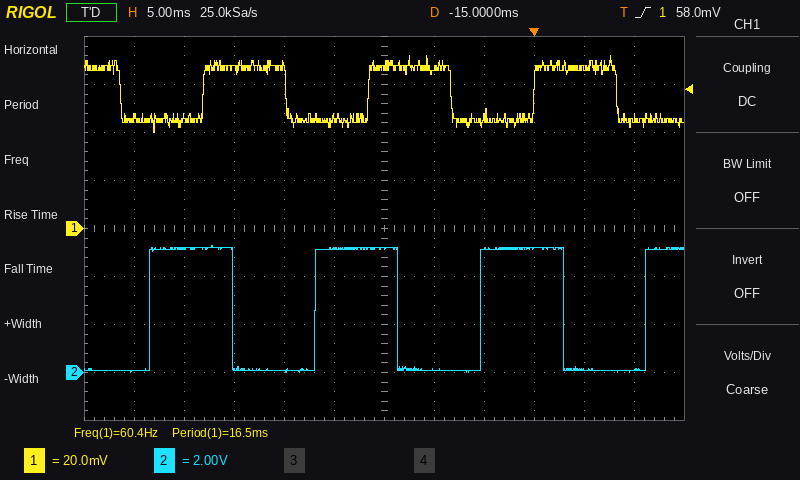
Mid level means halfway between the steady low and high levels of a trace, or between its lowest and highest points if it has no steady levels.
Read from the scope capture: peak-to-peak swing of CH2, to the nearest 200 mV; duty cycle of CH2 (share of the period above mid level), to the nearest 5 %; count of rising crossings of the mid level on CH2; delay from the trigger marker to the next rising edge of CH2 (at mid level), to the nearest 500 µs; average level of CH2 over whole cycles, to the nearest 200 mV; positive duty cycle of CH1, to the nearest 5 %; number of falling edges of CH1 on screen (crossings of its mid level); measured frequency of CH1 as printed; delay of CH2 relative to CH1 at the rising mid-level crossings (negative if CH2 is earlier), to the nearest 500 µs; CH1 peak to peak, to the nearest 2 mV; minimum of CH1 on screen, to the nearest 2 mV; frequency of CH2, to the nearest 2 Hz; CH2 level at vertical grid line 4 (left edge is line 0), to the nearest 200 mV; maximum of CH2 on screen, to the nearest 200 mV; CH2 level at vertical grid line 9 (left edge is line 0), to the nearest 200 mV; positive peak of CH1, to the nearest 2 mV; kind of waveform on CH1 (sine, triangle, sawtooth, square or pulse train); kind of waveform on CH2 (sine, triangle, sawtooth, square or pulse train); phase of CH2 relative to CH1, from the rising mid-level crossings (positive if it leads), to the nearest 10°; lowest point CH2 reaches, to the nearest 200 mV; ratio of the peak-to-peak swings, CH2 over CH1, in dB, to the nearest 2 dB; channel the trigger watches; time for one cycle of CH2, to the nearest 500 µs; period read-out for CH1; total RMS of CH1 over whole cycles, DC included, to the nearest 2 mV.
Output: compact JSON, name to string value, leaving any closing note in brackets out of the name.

{"peak-to-peak swing of CH2, to the nearest 200 mV": "5.2 V", "duty cycle of CH2 (share of the period above mid level), to the nearest 5 %": "50 %", "count of rising crossings of the mid level on CH2": "4", "delay from the trigger marker to the next rising edge of CH2 (at mid level), to the nearest 500 µs": "11.0 ms", "average level of CH2 over whole cycles, to the nearest 200 mV": "2.6 V", "positive duty cycle of CH1, to the nearest 5 %": "50 %", "number of falling edges of CH1 on screen": "4", "measured frequency of CH1 as printed": "60.4 Hz", "delay of CH2 relative to CH1 at the rising mid-level crossings (negative if CH2 is earlier), to the nearest 500 µs": "-5.5 ms", "CH1 peak to peak, to the nearest 2 mV": "32 mV", "minimum of CH1 on screen, to the nearest 2 mV": "40 mV", "frequency of CH2, to the nearest 2 Hz": "60 Hz", "CH2 level at vertical grid line 4 (left edge is line 0), to the nearest 200 mV": "0.0 V", "maximum of CH2 on screen, to the nearest 200 mV": "5.2 V", "CH2 level at vertical grid line 9 (left edge is line 0), to the nearest 200 mV": "5.2 V", "positive peak of CH1, to the nearest 2 mV": "72 mV", "kind of waveform on CH1": "square", "kind of waveform on CH2": "square", "phase of CH2 relative to CH1, from the rising mid-level crossings (positive if it leads), to the nearest 10°": "+120°", "lowest point CH2 reaches, to the nearest 200 mV": "0.0 V", "ratio of the peak-to-peak swings, CH2 over CH1, in dB, to the nearest 2 dB": "44 dB", "channel the trigger watches": "CH1", "time for one cycle of CH2, to the nearest 500 µs": "16.5 ms", "period read-out for CH1": "16.5 ms", "total RMS of CH1 over whole cycles, DC included, to the nearest 2 mV": "58 mV"}
